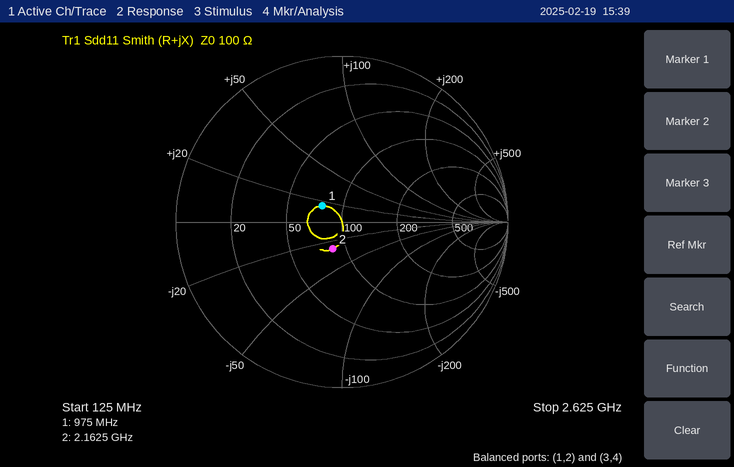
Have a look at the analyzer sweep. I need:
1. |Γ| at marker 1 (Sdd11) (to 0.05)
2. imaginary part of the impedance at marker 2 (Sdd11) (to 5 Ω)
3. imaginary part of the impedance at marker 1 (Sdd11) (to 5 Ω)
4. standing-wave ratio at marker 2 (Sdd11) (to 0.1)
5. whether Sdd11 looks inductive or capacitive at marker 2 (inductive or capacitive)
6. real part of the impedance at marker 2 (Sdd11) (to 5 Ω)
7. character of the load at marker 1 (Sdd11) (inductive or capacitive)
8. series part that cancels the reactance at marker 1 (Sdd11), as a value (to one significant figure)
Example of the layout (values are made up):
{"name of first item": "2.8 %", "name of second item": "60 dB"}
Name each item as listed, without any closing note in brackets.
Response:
{"|Γ| at marker 1 (Sdd11)": "0.15", "imaginary part of the impedance at marker 2 (Sdd11)": "-30 Ω", "imaginary part of the impedance at marker 1 (Sdd11)": "+15 Ω", "standing-wave ratio at marker 2 (Sdd11)": "1.4", "whether Sdd11 looks inductive or capacitive at marker 2": "capacitive", "real part of the impedance at marker 2 (Sdd11)": "85 Ω", "character of the load at marker 1 (Sdd11)": "inductive", "series part that cancels the reactance at marker 1 (Sdd11), as a value": "10 pF"}
